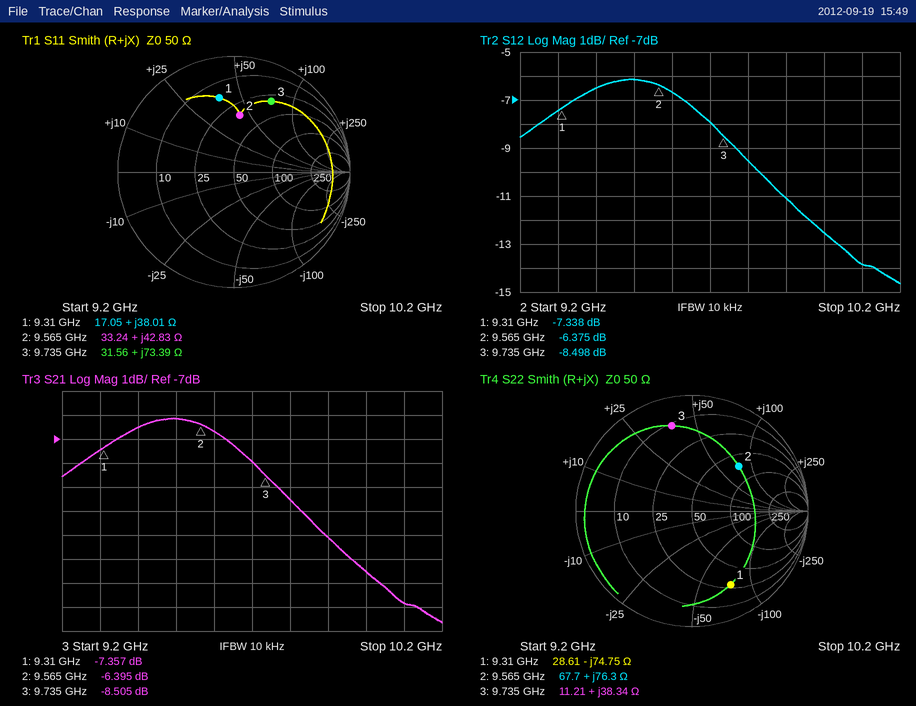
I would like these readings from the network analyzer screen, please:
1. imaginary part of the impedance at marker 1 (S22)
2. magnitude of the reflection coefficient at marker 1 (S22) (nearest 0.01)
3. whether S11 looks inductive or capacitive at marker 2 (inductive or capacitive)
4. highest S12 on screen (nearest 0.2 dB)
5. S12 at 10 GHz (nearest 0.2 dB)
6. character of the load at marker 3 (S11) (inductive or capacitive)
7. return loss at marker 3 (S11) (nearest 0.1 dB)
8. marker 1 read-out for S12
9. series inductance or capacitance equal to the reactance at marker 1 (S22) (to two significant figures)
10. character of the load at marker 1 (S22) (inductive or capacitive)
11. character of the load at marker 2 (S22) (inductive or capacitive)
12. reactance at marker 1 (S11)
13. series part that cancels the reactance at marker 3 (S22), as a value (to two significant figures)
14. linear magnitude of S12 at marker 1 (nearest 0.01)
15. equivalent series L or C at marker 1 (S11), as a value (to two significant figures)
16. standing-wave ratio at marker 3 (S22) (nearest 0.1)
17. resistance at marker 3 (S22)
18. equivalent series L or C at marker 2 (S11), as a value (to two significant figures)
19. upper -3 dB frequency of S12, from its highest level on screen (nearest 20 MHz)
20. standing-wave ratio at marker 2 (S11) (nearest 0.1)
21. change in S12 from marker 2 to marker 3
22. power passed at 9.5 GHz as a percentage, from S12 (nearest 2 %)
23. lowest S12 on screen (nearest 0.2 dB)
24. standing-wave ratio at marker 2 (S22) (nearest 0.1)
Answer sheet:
-74.75 Ω
0.72
inductive
-6.2 dB
-12.6 dB
inductive
3.2 dB
-7.338 dB
230 fF
capacitive
inductive
+38.01 Ω
430 fF
0.43
650 pH
7.2
11.21 Ω
710 pH
9.78 GHz
2.9
-2.123 dB
24 %
-14.6 dB
3.5
